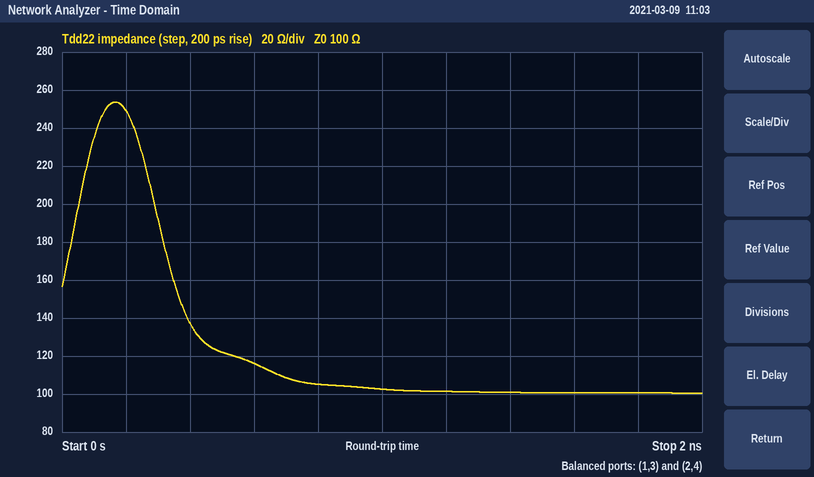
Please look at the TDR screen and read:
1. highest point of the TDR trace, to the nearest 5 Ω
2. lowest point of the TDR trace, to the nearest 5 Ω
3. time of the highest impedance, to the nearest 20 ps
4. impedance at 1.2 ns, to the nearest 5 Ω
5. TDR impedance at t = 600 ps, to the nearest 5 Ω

255 Ω
100 Ω
160 ps
100 Ω
115 Ω
